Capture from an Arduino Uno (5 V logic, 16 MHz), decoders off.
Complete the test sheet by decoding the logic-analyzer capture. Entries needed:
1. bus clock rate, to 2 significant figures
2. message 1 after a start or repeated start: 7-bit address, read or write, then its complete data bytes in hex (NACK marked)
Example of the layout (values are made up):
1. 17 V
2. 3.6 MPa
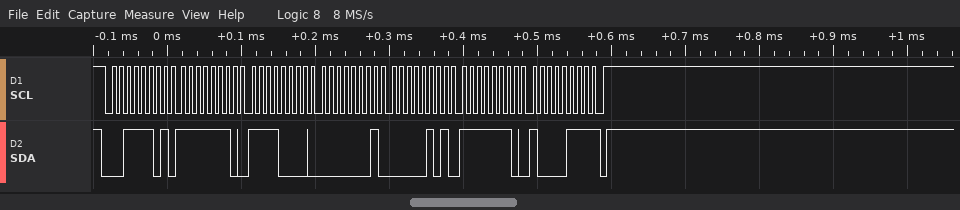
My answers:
1. 100 kHz
2. 0x1E read: FE F0 01 05 FE 87 NACK
